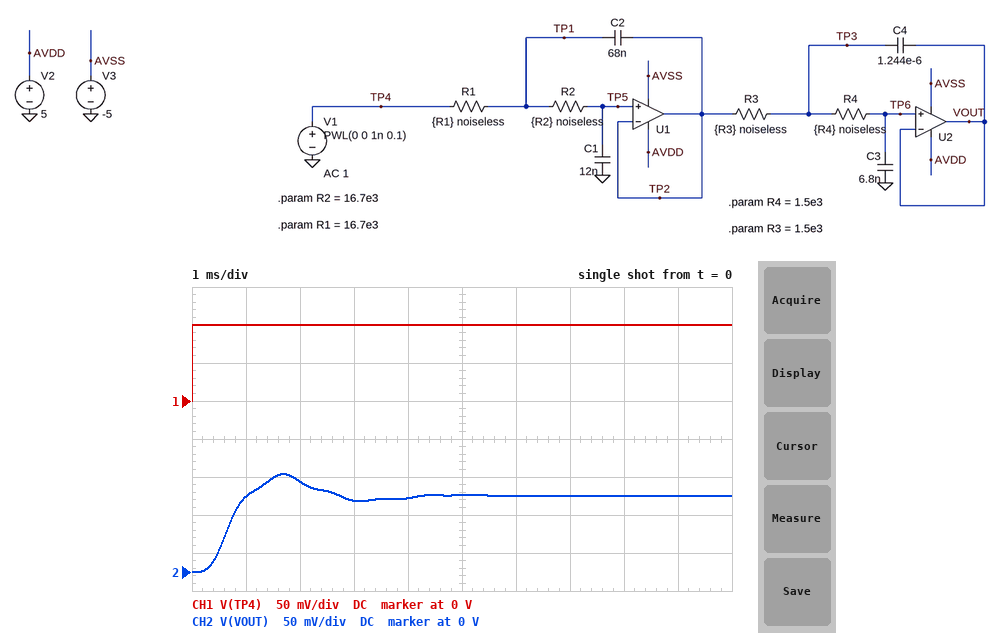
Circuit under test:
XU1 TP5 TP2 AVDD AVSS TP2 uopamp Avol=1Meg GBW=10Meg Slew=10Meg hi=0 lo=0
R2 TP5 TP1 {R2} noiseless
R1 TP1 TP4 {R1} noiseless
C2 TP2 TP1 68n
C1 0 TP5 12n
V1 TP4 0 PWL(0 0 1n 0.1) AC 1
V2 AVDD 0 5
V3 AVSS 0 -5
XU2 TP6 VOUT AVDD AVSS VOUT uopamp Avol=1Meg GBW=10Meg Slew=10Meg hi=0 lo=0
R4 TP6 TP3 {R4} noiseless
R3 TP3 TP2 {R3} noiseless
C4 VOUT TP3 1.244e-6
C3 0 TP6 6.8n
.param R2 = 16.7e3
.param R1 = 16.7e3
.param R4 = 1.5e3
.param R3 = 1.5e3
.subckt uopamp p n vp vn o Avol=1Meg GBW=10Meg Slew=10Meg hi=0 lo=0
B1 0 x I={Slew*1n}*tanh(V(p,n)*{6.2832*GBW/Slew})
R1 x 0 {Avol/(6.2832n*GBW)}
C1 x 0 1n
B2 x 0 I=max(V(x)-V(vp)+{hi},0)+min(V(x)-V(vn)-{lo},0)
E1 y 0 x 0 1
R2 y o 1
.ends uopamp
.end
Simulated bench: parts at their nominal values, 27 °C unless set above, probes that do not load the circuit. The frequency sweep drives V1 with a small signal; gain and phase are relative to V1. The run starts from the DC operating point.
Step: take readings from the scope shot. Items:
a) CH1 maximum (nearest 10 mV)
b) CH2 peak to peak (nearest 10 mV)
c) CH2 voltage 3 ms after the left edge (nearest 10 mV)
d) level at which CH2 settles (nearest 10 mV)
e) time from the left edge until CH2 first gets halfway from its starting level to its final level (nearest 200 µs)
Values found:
100 mV
130 mV
90 mV
100 mV
600 µs
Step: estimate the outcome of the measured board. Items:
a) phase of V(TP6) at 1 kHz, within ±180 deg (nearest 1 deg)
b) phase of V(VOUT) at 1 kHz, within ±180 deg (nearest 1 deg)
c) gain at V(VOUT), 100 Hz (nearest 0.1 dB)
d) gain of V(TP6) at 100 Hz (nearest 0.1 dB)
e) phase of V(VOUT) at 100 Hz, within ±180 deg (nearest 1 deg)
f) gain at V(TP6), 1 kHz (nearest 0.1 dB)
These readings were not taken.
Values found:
170 deg
170 deg
0.6 dB
0.6 dB
-16 deg
-7.4 dB
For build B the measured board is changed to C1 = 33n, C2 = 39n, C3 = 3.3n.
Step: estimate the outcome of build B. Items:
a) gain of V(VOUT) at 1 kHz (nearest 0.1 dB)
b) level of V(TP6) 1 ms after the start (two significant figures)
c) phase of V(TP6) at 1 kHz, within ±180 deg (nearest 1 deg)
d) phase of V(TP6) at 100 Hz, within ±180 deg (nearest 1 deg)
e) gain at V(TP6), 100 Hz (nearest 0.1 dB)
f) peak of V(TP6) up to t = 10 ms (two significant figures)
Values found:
-19.5 dB
51 mV
-158 deg
-39 deg
-0.8 dB
100 mV
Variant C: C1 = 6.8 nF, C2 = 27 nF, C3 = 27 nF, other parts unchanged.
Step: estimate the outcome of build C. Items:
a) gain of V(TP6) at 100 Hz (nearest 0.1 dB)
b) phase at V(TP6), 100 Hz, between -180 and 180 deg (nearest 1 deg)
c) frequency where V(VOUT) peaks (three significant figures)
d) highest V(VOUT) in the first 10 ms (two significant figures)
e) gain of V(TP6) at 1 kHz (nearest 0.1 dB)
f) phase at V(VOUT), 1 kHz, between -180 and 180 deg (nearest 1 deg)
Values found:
0.3 dB
-11 deg
563 Hz
170 mV
-11.1 dB
69 deg
